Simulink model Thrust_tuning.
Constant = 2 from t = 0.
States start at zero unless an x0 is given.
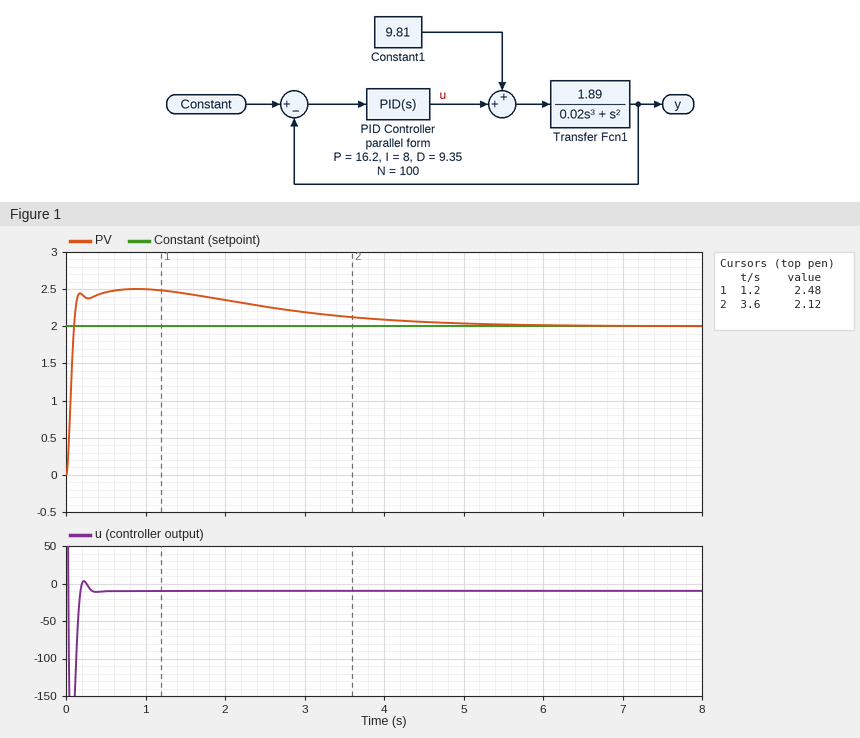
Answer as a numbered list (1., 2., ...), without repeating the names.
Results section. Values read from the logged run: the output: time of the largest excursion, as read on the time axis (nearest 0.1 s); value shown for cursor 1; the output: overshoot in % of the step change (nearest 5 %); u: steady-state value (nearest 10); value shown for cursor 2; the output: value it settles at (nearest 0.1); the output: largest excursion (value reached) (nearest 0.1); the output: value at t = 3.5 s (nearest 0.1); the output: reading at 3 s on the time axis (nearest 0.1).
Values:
1. 0.9 s
2. 2.48
3. 25 %
4. -10
5. 2.12
6. 2.0
7. 2.5
8. 2.1
9. 2.2
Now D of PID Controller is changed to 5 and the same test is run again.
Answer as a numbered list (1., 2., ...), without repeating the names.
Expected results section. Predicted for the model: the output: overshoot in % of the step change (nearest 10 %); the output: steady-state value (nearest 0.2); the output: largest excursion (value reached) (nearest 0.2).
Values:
1. 40 %
2. 2.0
3. 2.8
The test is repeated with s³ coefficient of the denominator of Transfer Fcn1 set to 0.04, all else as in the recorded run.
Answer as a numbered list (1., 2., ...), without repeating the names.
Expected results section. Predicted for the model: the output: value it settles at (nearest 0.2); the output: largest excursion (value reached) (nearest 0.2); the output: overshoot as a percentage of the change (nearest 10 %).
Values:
1. 2.0
2. 2.8
3. 40 %
